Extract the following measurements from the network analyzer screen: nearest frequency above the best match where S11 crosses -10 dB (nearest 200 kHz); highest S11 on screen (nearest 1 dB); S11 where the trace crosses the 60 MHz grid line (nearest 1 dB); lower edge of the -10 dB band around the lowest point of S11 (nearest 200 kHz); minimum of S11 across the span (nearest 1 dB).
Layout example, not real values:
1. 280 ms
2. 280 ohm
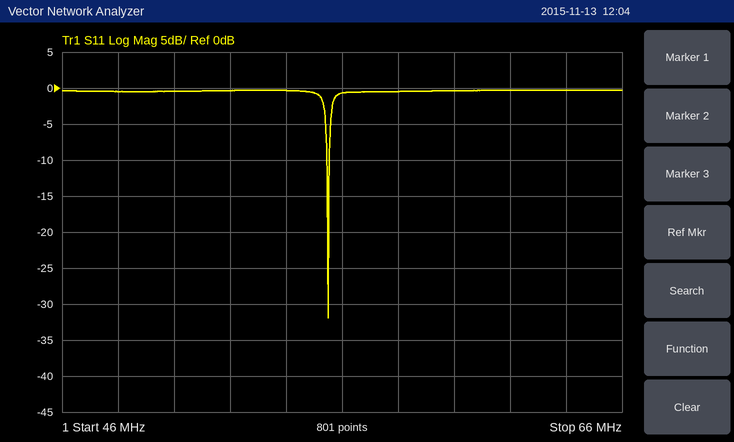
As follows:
1. 55.6 MHz
2. 0 dB
3. 0 dB
4. 55.4 MHz
5. -32 dB
